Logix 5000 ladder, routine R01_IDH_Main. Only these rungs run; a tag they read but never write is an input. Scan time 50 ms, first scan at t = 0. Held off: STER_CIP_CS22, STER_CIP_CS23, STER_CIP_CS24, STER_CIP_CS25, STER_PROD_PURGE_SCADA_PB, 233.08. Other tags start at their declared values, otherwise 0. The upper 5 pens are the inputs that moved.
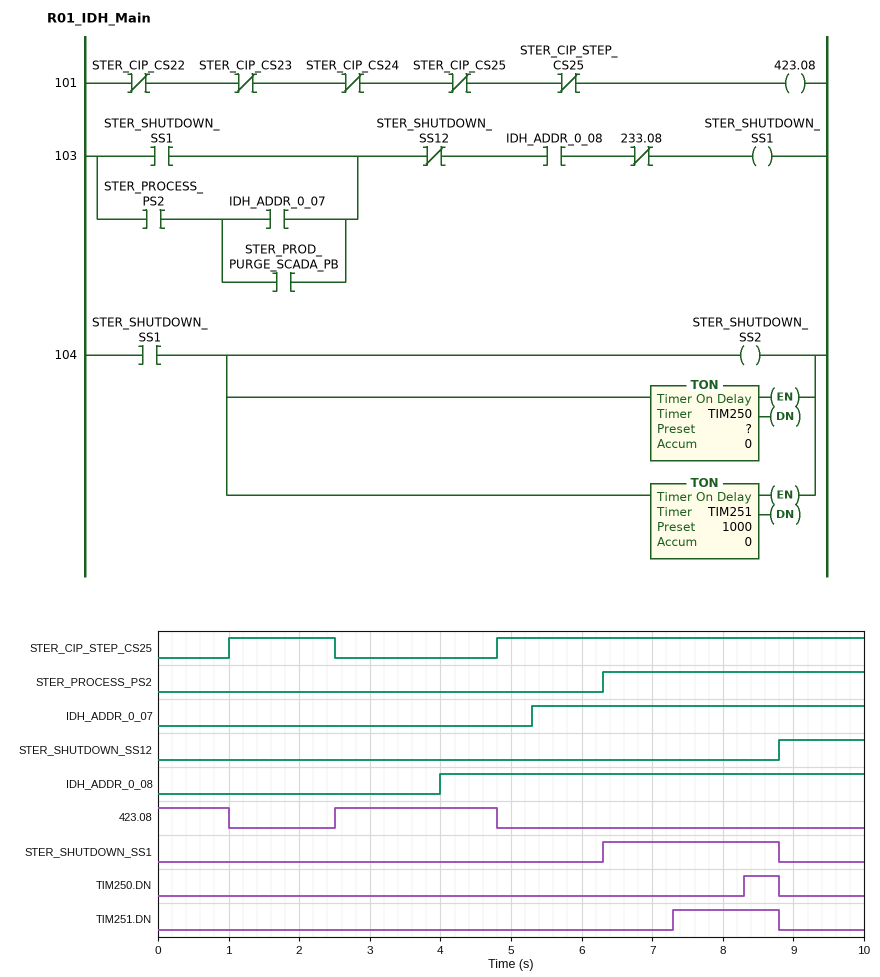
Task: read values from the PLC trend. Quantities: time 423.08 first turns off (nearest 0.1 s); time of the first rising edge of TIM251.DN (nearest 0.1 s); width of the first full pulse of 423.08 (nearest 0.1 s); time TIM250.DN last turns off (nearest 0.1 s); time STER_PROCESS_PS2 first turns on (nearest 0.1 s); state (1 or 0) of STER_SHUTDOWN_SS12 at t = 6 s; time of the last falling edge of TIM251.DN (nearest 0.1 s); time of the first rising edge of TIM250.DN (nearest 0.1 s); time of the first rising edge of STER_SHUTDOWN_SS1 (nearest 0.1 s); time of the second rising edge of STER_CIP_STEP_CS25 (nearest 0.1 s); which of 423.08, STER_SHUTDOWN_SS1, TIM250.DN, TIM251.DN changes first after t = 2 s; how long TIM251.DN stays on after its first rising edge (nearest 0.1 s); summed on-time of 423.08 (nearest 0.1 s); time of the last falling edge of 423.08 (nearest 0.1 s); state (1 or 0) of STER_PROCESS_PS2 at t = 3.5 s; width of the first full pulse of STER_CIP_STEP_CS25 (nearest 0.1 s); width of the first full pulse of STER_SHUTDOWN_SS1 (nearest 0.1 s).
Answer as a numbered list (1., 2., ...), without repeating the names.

1. 1.0 s
2. 7.3 s
3. 2.3 s
4. 8.8 s
5. 6.3 s
6. 0
7. 8.8 s
8. 8.3 s
9. 6.3 s
10. 4.8 s
11. 423.08
12. 1.5 s
13. 3.3 s
14. 4.8 s
15. 0
16. 1.5 s
17. 2.5 s
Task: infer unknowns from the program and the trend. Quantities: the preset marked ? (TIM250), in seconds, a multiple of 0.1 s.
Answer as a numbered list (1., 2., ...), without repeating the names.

1. 2.0 s
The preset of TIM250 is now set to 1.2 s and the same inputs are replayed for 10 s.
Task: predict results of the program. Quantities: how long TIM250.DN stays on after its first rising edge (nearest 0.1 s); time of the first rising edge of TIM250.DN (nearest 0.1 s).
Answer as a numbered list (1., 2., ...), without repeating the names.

1. 1.3 s
2. 7.5 s
